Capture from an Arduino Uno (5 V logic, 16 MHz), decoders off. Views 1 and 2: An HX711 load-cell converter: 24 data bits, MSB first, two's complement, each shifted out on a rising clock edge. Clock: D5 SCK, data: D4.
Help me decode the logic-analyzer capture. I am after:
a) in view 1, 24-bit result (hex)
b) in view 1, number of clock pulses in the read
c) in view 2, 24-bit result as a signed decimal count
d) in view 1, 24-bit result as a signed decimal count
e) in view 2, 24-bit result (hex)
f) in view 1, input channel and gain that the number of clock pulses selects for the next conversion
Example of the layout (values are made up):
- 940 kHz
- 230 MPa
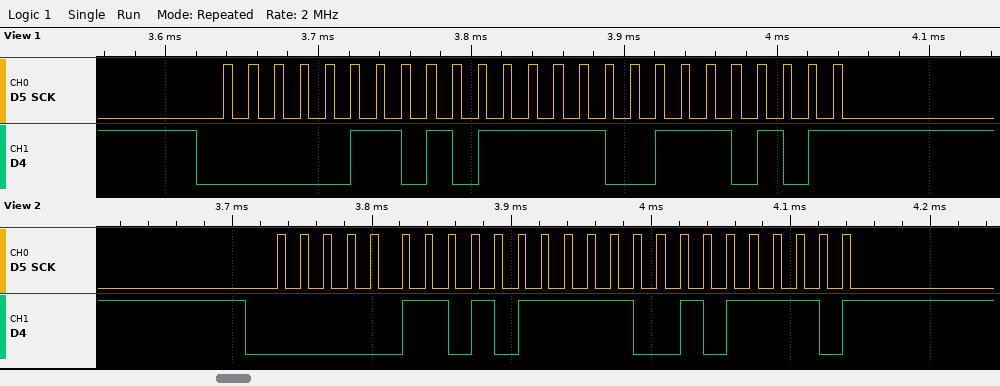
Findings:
- 0x06BE75
- 25
- 441950
- 441973
- 0x06BE5E
- channel A, gain 128
